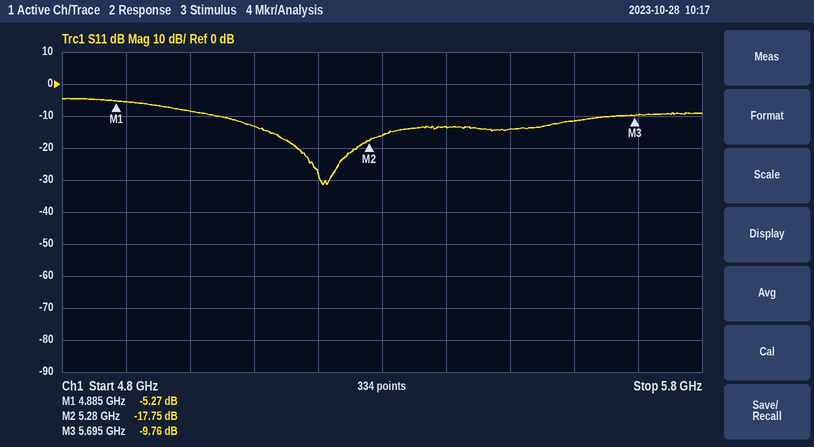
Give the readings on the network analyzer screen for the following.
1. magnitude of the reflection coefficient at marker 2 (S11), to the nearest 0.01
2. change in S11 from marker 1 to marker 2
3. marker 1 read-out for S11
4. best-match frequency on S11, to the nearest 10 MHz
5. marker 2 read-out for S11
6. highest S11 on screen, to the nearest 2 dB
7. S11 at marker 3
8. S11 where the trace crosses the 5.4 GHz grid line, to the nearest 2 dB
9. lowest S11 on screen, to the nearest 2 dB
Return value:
0.13
-12.48 dB
-5.27 dB
5.21 GHz
-17.75 dB
-4 dB
-9.76 dB
-14 dB
-32 dB
